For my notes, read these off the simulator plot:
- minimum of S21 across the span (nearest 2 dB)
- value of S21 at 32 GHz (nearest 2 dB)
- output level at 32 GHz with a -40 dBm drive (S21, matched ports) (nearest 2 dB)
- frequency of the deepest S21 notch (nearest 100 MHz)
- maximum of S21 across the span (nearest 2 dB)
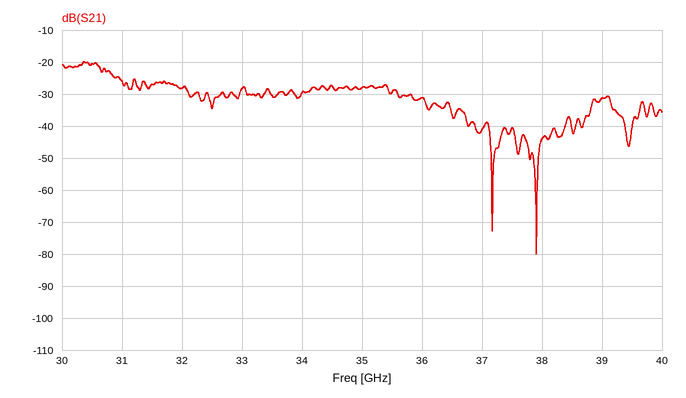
-80 dB
-28 dB
-68 dBm
37.9 GHz
-20 dB
